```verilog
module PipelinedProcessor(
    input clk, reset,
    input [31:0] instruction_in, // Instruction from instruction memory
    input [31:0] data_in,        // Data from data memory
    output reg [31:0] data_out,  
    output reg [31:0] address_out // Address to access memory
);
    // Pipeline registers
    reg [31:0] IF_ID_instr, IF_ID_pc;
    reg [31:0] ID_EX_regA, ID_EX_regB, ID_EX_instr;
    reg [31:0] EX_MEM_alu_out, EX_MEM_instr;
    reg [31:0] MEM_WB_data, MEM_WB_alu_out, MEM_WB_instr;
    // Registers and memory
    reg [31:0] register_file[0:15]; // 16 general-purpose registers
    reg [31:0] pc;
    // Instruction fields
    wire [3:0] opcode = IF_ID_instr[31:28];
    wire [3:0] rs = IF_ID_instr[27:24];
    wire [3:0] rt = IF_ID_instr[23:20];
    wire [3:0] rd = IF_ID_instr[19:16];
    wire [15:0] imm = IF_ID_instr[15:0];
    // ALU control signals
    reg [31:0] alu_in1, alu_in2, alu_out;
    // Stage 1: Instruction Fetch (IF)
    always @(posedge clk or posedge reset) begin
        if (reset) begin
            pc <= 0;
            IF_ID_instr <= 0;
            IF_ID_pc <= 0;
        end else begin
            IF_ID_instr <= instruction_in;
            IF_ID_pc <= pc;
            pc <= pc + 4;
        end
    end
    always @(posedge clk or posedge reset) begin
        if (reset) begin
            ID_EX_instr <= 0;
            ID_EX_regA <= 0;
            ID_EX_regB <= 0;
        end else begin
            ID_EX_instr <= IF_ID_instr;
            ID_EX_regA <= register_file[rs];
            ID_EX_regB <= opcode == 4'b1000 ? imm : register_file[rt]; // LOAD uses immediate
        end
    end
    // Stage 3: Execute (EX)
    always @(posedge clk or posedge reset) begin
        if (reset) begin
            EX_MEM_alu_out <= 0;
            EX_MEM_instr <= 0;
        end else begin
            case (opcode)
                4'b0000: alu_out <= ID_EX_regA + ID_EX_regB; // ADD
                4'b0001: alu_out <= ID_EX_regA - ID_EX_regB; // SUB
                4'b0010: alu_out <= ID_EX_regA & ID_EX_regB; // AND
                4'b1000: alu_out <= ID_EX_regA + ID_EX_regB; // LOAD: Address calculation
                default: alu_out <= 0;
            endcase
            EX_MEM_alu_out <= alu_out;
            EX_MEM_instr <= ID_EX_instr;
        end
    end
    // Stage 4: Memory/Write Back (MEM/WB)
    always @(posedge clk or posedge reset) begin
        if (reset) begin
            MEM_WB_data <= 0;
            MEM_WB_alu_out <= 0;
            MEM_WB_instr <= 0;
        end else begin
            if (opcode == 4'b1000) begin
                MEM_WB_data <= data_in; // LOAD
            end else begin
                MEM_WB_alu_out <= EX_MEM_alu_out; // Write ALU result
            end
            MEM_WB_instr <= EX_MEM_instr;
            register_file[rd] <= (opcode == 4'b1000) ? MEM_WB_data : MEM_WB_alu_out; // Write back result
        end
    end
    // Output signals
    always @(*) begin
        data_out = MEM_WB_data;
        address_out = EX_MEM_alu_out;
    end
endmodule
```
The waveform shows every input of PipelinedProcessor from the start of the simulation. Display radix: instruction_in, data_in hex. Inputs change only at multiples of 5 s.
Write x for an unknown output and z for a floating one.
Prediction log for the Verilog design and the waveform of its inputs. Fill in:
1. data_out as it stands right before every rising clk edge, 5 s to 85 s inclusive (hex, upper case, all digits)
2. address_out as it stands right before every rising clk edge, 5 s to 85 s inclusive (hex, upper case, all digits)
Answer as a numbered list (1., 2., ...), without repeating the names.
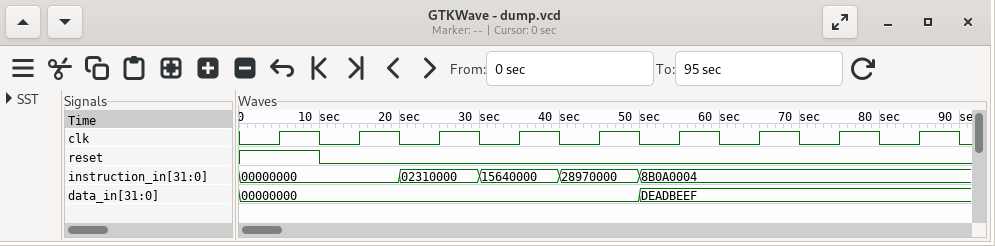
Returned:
1. 00000000, 00000000, 00000000, 00000000, 00000000, 00000000, 00000000, DEADBEEF, DEADBEEF
2. 00000000, 00000000, x, 00000000, x, 00000000, x, x, x
